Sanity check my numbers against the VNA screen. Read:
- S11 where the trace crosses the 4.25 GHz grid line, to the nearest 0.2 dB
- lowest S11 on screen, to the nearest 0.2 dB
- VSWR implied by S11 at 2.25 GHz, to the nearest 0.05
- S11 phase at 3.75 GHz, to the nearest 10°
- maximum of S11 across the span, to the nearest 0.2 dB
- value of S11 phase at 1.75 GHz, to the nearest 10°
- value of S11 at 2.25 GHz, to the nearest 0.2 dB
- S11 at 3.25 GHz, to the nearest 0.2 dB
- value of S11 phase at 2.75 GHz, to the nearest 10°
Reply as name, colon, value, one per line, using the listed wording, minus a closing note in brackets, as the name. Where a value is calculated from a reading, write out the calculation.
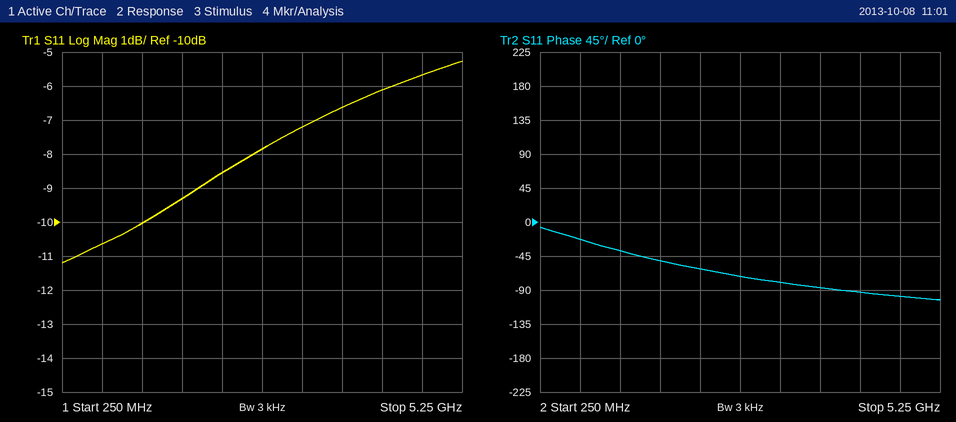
S11 where the trace crosses the 4.25 GHz grid line, to the nearest 0.2 dB: -6.2 dB
lowest S11 on screen, to the nearest 0.2 dB: -11.2 dB
VSWR implied by S11 at 2.25 GHz, to the nearest 0.05: |Γ| = 10^(-8.6/20) = 0.3715; VSWR = (1 + 0.3715)/(1 − 0.3715) ≈ 2.18, so 2.20 to the nearest 0.05
S11 phase at 3.75 GHz, to the nearest 10°: -90°
maximum of S11 across the span, to the nearest 0.2 dB: -5.2 dB
value of S11 phase at 1.75 GHz, to the nearest 10°: -50°
value of S11 at 2.25 GHz, to the nearest 0.2 dB: -8.6 dB
S11 at 3.25 GHz, to the nearest 0.2 dB: -7.2 dB
value of S11 phase at 2.75 GHz, to the nearest 10°: -70°
